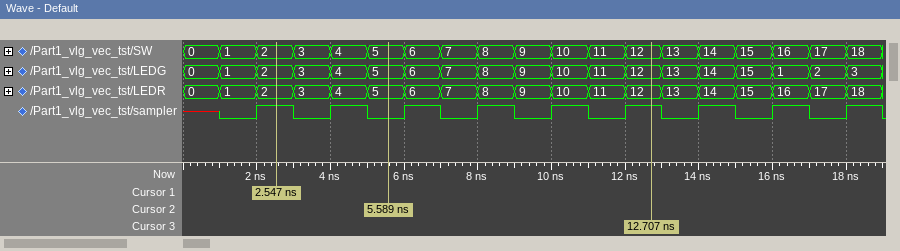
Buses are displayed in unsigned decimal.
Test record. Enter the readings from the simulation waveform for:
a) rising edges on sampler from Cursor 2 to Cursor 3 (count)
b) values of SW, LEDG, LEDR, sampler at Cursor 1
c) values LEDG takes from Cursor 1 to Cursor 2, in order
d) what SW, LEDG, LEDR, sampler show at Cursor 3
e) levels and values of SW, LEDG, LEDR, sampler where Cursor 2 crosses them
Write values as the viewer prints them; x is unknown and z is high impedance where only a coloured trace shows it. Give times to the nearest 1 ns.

4
SW=2, LEDG=2, LEDR=2, sampler=1
2, 3, 4, 5
SW=12, LEDG=12, LEDR=12, sampler=1
SW=5, LEDG=5, LEDR=5, sampler=0
